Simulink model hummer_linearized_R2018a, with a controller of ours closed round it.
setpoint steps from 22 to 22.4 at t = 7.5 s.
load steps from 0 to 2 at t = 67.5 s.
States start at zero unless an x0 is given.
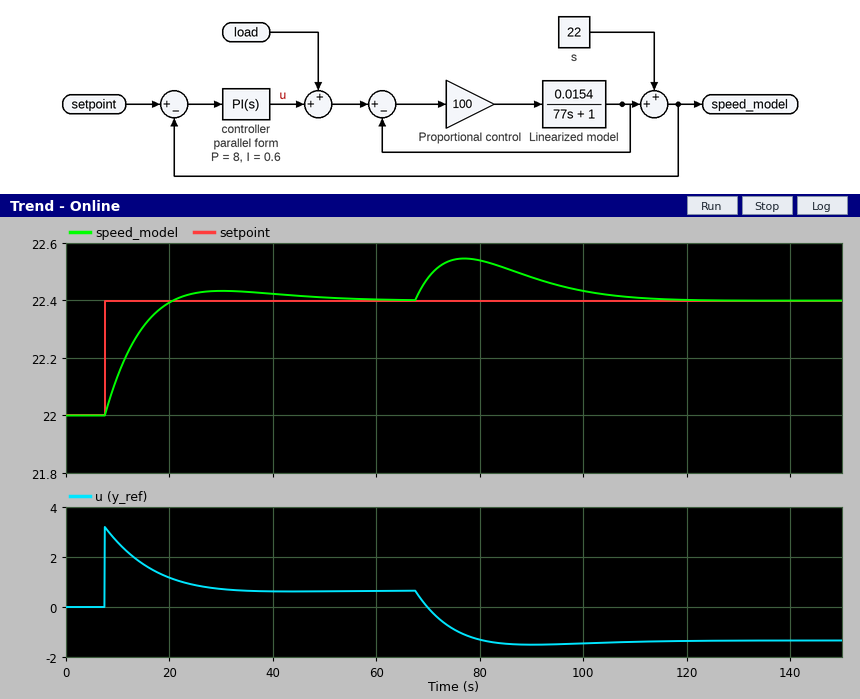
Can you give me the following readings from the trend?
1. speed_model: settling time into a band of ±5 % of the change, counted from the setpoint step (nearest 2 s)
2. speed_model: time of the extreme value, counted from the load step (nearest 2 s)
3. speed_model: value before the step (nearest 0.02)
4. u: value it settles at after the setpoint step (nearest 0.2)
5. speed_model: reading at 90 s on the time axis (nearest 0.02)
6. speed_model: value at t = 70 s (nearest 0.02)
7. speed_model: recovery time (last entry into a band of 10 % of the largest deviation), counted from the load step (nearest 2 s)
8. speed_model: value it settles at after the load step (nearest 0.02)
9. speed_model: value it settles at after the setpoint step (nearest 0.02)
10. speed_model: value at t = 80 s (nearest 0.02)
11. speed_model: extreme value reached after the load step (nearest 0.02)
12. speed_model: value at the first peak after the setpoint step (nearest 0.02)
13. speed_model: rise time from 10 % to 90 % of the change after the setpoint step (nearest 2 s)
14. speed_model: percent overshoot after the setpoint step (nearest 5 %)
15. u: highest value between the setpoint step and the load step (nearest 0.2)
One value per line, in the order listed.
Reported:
34 s
10 s
22.00
0.6
22.48
22.48
40 s
22.40
22.40
22.54
22.54
22.44
10 s
10 %
3.2
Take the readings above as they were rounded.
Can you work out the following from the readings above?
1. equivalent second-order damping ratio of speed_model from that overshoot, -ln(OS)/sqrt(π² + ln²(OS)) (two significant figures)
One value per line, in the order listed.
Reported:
0.59
